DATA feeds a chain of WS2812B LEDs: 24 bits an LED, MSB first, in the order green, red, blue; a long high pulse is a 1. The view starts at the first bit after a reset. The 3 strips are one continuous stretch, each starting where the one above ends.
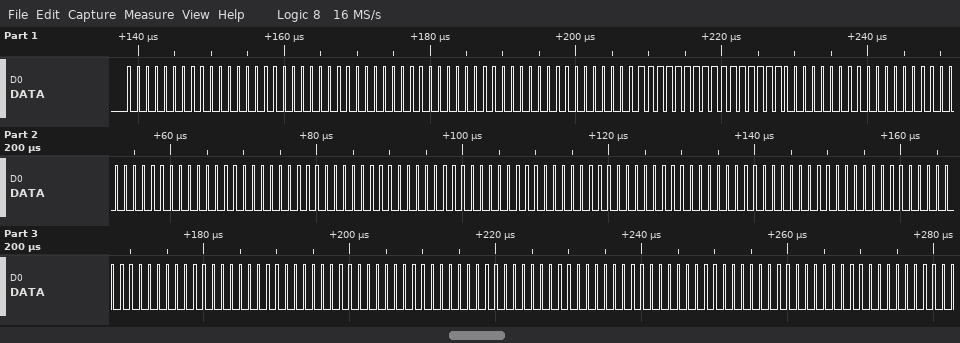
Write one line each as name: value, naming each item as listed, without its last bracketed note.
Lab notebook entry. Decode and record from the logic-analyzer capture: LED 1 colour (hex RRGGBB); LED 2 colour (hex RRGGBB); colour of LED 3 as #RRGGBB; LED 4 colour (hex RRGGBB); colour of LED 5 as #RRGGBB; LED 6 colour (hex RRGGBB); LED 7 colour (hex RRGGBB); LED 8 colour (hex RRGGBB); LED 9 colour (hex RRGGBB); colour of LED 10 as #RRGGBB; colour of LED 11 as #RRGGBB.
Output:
LED 1 colour: #000000
LED 2 colour: #000000
colour of LED 3 as #RRGGBB: #FF00FF
LED 4 colour: #000000
colour of LED 5 as #RRGGBB: #000000
LED 6 colour: #000000
LED 7 colour: #000000
LED 8 colour: #000000
LED 9 colour: #000000
colour of LED 10 as #RRGGBB: #000000
colour of LED 11 as #RRGGBB: #000000
